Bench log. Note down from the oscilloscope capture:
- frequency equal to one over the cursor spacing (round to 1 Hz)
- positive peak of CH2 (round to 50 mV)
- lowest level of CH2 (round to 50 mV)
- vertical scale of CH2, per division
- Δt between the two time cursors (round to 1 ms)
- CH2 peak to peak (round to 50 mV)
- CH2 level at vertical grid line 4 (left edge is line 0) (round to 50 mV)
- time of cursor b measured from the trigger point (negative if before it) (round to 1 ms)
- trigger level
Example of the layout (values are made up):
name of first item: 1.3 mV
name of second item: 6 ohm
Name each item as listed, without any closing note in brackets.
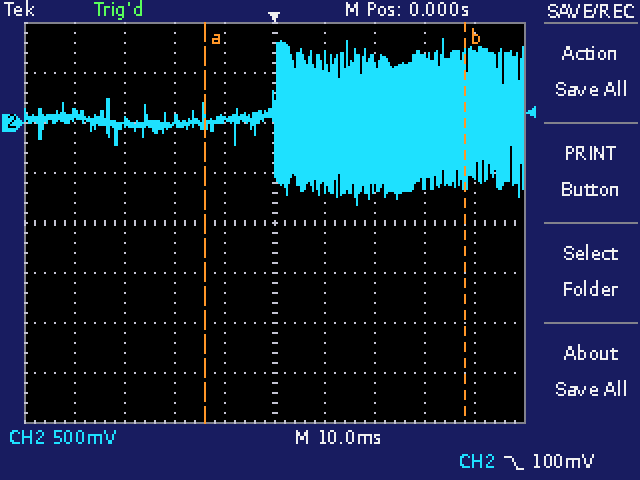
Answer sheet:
frequency equal to one over the cursor spacing: 19 Hz
positive peak of CH2: 850 mV
lowest level of CH2: -800 mV
vertical scale of CH2, per division: 500 mV
Δt between the two time cursors: 52 ms
CH2 peak to peak: 1.65 V
CH2 level at vertical grid line 4 (left edge is line 0): 50 mV
time of cursor b measured from the trigger point (negative if before it): +38 ms
trigger level: 100 mV
